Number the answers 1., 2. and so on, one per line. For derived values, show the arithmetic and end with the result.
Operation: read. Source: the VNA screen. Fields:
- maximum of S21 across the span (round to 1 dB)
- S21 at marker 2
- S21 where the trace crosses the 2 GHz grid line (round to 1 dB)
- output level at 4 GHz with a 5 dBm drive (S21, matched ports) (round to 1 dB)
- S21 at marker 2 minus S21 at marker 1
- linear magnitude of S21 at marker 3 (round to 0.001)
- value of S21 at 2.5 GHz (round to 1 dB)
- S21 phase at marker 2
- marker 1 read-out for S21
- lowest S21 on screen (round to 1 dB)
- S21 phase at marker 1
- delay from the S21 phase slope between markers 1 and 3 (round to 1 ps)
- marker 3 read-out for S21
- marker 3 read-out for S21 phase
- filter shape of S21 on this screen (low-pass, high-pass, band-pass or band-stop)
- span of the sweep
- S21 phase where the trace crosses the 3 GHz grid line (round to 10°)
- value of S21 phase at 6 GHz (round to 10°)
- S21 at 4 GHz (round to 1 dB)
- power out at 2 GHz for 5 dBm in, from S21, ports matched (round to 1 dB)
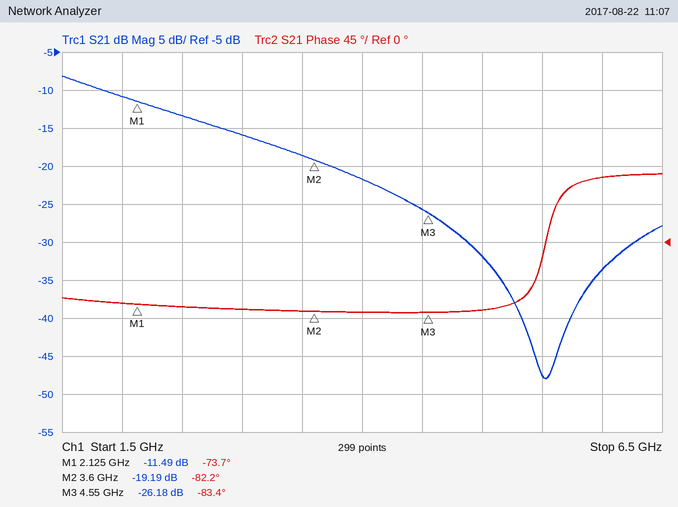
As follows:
1. -8 dB
2. -19.19 dB
3. -11 dB
4. 5 dBm + (-22 dB) = -17 dBm
5. -19.19 − (-11.49) = -7.70 dB
6. 10^(-26.18/20) ≈ 0.049
7. -13 dB
8. -82.2°
9. -11.49 dB
10. -48 dB
11. -73.7°
12. −(-83.4° − (-73.7°))/(360° × 2.425 GHz) ≈ 11 ps
13. -26.18 dB
14. -83.4°
15. low-pass
16. 5 GHz
17. -80°
18. 80°
19. -22 dB
20. 5 dBm + (-11 dB) = -6 dBm
